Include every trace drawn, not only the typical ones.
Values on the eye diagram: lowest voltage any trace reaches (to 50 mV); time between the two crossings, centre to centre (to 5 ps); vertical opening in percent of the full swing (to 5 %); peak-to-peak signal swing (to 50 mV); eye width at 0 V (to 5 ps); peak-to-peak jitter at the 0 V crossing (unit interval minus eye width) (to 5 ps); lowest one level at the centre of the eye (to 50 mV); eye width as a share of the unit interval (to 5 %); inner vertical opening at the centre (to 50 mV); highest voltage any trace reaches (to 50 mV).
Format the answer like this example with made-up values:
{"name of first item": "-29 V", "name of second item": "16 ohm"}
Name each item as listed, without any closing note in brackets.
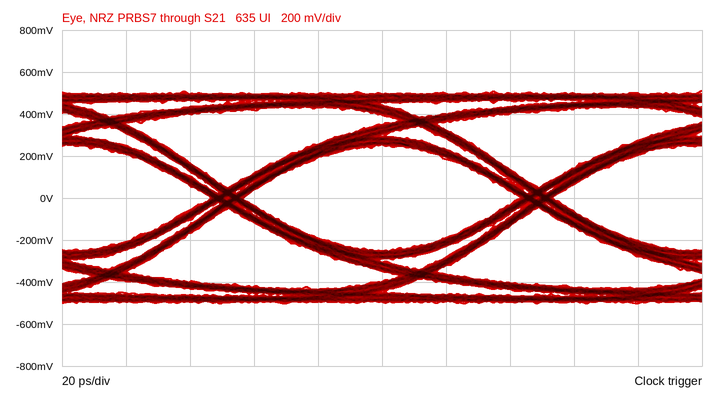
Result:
{"lowest voltage any trace reaches": "-500 mV", "time between the two crossings, centre to centre": "95 ps", "vertical opening in percent of the full swing": "50 %", "peak-to-peak signal swing": "1.00 V", "eye width at 0 V": "85 ps", "peak-to-peak jitter at the 0 V crossing (unit interval minus eye width)": "10 ps", "lowest one level at the centre of the eye": "250 mV", "eye width as a share of the unit interval": "90 %", "inner vertical opening at the centre": "500 mV", "highest voltage any trace reaches": "500 mV"}
